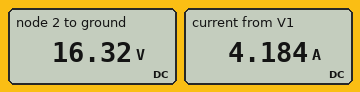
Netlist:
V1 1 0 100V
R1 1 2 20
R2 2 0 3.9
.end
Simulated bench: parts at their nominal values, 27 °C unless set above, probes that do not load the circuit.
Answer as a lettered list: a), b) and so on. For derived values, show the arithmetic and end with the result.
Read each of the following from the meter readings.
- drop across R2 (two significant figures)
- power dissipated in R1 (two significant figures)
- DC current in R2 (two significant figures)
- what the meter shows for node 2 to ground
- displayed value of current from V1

a) 16.32 V = 16 V
b) (100 V - 16.32 V)^2 / 20 Ω = 350 W
c) (16.32 V) / 3.9 Ω = 4.2 A
d) 16.32 V
e) 4.184 A
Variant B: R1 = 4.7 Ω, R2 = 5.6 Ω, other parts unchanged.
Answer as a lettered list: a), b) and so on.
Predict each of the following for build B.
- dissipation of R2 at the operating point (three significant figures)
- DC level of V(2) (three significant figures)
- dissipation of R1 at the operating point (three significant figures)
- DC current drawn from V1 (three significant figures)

a) 528 W
b) 54.4 V
c) 443 W
d) 9.71 A
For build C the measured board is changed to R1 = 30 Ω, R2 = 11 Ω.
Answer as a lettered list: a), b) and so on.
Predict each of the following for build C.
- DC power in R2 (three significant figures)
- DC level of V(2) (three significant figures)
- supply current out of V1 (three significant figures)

a) 65.4 W
b) 26.8 V
c) 2.44 A
